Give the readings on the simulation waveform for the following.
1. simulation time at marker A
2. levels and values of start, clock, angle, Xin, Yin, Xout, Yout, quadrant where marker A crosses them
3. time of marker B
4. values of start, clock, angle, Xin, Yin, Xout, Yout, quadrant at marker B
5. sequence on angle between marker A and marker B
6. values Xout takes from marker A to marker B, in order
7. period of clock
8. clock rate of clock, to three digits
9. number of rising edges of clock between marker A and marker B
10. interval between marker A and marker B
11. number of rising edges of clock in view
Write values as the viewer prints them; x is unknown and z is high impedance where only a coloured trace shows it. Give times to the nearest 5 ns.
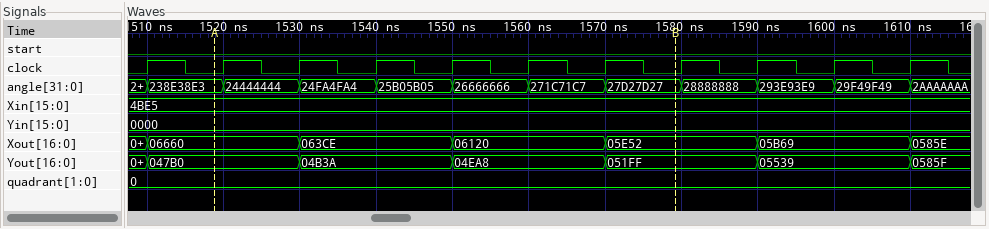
1520 ns
start=0, clock=0, angle=238E38E3, Xin=4BE5, Yin=0000, Xout=06660, Yout=047B0, quadrant=0
1580 ns
start=0, clock=0, angle=27D27D27, Xin=4BE5, Yin=0000, Xout=05E52, Yout=051FF, quadrant=0
238E38E3, 24444444, 24FA4FA4, 25B05B05, 26666666, 271C71C7, 27D27D27
06660, 063CE, 06120, 05E52
10 ns
100 MHz
6
60 ns
11
